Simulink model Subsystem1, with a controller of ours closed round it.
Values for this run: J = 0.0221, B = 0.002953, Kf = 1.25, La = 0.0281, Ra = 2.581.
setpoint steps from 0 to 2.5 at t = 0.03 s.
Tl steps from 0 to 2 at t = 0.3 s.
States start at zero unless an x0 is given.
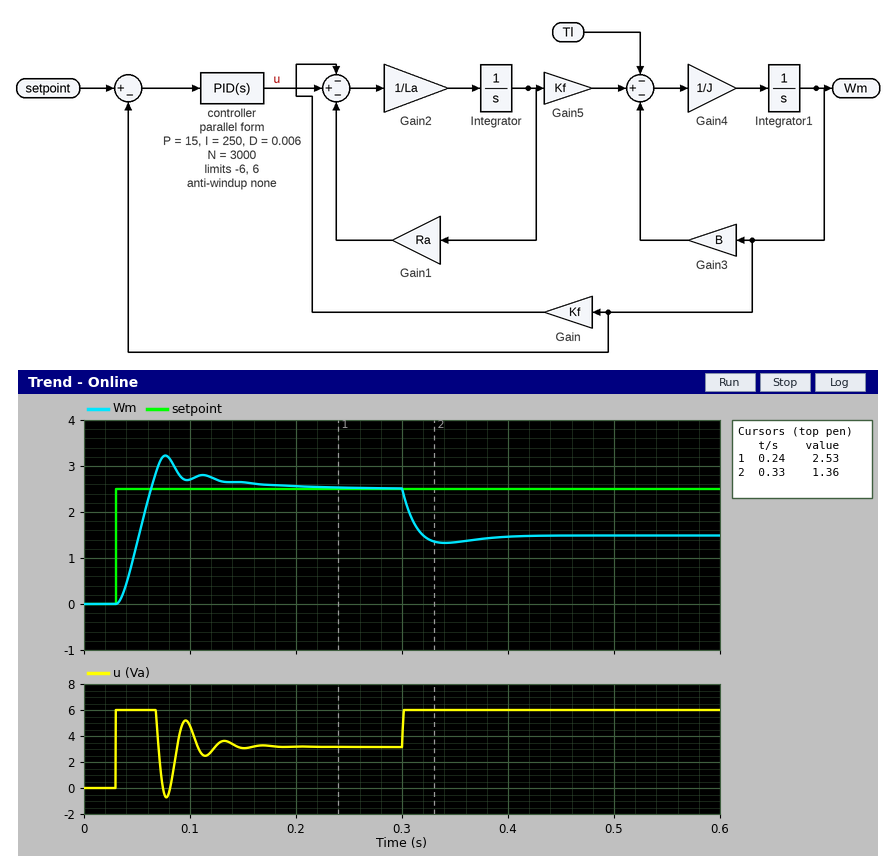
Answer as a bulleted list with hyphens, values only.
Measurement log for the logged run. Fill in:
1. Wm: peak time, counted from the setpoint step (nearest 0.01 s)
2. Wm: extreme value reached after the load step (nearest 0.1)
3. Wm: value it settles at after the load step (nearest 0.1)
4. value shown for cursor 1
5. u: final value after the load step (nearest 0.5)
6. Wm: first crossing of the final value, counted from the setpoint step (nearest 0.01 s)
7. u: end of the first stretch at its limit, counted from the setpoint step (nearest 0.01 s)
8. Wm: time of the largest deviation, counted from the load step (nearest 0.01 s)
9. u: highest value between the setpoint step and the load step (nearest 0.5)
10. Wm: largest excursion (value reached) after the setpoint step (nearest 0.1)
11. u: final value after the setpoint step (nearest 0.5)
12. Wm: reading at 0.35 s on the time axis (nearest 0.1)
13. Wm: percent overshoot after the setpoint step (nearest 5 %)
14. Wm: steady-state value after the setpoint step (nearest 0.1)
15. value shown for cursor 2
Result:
- 0.05 s
- 1.3
- 1.5
- 2.53
- 6.0
- 0.03 s
- 0.04 s
- 0.04 s
- 6.0
- 3.2
- 3.0
- 1.3
- 30 %
- 2.5
- 1.36
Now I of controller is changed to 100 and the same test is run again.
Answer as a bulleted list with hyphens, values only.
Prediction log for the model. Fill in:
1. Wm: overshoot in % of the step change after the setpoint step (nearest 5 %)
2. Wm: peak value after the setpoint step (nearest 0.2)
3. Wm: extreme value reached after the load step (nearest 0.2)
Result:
- 15 %
- 2.8
- 1.4
